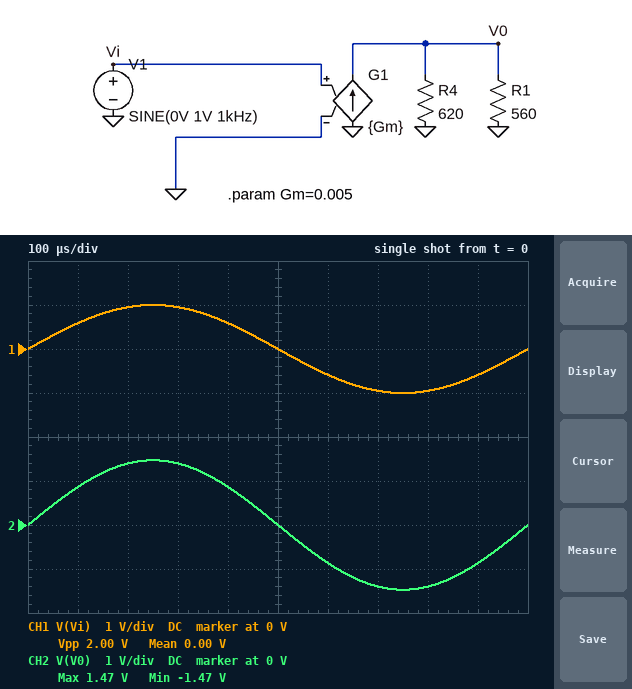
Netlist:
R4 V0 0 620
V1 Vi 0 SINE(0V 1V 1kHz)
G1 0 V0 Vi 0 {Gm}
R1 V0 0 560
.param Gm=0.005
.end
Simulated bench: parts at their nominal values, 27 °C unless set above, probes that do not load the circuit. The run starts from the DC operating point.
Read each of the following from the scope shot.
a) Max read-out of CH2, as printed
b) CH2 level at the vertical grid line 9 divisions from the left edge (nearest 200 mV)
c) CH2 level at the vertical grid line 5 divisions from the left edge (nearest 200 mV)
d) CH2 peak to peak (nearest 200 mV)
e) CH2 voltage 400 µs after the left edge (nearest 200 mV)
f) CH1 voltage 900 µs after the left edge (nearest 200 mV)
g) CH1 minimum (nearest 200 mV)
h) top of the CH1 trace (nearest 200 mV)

1.47 V
-800 mV
0 V
3.0 V
800 mV
-600 mV
-1.0 V
1.0 V
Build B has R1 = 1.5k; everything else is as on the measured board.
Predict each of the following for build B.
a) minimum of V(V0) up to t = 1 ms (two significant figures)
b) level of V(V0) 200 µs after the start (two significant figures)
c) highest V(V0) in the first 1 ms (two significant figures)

-2.2 V
2.1 V
2.2 V
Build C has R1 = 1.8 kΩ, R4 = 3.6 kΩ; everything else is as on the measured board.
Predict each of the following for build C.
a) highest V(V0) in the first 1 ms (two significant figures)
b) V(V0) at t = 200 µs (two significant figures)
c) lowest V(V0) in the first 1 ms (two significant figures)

6.0 V
5.7 V
-6.0 V
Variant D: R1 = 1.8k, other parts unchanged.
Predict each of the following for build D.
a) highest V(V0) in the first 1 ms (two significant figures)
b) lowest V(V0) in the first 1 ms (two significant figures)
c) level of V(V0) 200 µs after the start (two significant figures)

2.3 V
-2.3 V
2.2 V
